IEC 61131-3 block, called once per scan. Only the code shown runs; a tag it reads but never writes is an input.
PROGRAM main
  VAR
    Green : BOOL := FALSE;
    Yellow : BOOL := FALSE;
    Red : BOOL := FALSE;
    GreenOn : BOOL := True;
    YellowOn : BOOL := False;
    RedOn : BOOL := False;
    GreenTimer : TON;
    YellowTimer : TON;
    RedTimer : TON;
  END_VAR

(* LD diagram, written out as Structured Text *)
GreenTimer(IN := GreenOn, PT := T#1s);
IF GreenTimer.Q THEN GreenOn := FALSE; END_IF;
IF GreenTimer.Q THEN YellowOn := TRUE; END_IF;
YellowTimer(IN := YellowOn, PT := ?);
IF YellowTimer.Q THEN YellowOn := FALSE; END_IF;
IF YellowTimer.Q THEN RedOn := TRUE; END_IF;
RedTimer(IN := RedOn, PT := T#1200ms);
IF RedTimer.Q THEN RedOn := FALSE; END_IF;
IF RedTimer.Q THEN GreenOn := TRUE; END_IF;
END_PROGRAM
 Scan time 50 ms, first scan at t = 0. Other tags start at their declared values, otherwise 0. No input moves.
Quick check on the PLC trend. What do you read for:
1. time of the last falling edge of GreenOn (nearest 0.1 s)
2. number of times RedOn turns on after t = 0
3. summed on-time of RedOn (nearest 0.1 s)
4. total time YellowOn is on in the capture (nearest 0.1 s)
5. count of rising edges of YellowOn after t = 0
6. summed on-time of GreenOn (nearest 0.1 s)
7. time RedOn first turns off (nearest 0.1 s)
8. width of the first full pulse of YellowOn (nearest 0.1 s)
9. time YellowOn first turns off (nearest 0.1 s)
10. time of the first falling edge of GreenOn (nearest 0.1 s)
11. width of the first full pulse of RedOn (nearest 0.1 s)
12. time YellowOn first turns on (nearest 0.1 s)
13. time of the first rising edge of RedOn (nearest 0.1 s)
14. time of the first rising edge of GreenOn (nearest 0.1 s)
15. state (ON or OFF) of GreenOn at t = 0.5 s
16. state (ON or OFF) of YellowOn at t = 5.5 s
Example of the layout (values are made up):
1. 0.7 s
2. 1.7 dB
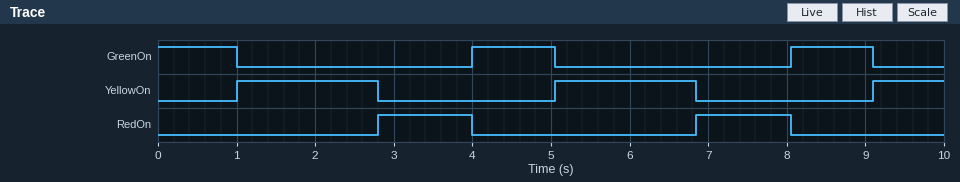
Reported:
1. 9.1 s
2. 2
3. 2.4 s
4. 4.5 s
5. 3
6. 3.1 s
7. 4.0 s
8. 1.8 s
9. 2.8 s
10. 1.0 s
11. 1.2 s
12. 1.0 s
13. 2.8 s
14. 4.0 s
15. ON
16. ON
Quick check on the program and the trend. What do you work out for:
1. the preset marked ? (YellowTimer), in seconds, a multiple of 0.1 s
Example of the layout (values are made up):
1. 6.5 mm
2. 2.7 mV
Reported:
1. 1.8 s
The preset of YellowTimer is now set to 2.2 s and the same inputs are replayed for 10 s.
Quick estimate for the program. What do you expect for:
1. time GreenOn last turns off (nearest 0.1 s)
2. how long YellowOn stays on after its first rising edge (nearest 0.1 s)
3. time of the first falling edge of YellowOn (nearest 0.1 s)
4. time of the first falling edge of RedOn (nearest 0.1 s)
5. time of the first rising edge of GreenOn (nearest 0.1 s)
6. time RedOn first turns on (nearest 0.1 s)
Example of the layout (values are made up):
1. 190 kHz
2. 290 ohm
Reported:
1. 9.9 s
2. 2.2 s
3. 3.2 s
4. 4.4 s
5. 4.4 s
6. 3.2 s
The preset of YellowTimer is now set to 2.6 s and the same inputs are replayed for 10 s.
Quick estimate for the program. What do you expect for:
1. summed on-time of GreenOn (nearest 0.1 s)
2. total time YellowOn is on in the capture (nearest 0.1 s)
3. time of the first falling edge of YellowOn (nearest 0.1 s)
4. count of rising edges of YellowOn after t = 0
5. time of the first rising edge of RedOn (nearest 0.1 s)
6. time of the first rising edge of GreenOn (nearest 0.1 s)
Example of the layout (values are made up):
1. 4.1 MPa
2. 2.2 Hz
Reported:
1. 2.4 s
2. 5.2 s
3. 3.6 s
4. 2
5. 3.6 s
6. 4.8 s
